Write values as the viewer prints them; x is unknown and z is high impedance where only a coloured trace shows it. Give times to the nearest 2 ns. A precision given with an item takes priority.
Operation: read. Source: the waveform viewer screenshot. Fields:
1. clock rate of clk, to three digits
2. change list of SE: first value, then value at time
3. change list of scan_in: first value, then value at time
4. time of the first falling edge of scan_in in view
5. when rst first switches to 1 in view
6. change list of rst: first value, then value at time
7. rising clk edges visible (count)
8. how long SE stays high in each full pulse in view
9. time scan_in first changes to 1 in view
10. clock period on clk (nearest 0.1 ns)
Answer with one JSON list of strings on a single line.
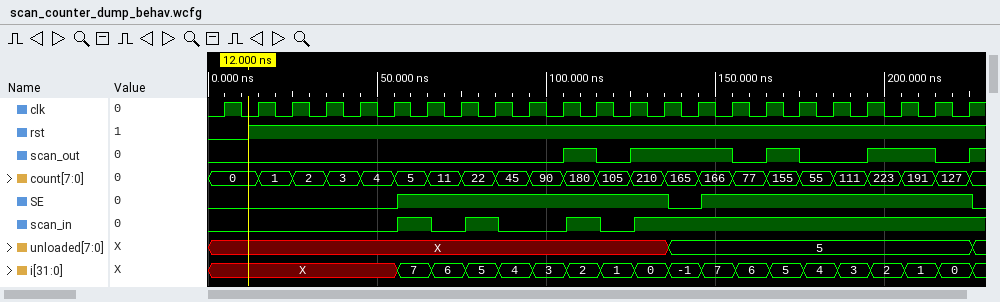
["100 MHz", "0, 1 at 56 ns, 0 at 136 ns, 1 at 146 ns, 0 at 226 ns", "0, 1 at 56 ns, 0 at 66 ns, 1 at 76 ns, 0 at 86 ns, 1 at 106 ns, 0 at 116 ns, 1 at 126 ns", "66 ns", "12 ns", "0, 1 at 12 ns", "23", "80 ns, 80 ns", "56 ns", "10 ns"]
